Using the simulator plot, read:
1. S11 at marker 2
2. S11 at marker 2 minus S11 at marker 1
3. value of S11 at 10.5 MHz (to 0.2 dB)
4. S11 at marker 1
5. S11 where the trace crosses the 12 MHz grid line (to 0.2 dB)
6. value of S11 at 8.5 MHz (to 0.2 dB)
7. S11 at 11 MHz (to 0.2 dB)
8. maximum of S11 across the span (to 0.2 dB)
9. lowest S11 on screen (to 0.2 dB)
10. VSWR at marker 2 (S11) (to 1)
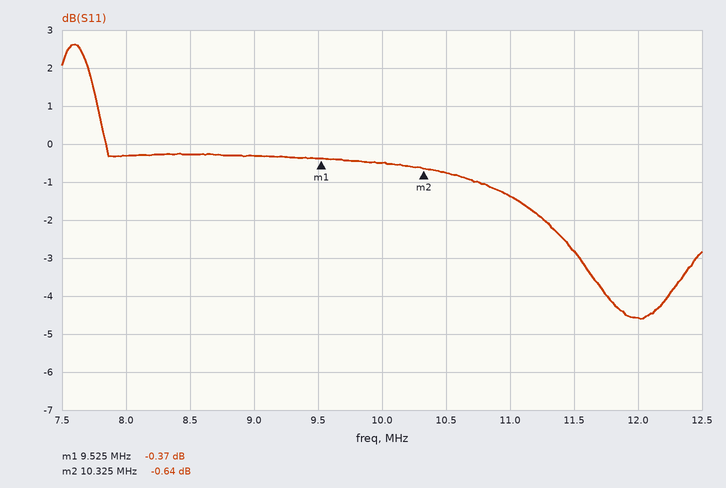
-0.64 dB
-0.27 dB
-0.8 dB
-0.37 dB
-4.6 dB
-0.2 dB
-1.4 dB
2.6 dB
-4.6 dB
27
